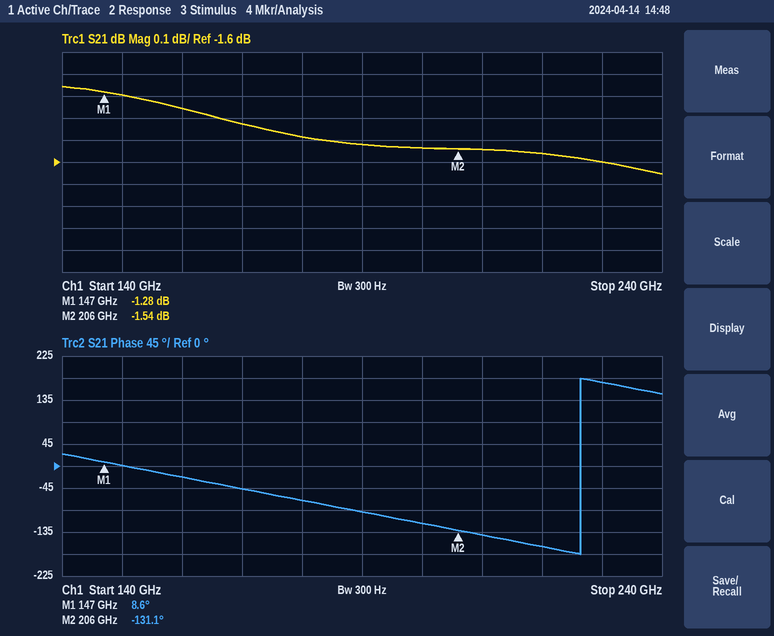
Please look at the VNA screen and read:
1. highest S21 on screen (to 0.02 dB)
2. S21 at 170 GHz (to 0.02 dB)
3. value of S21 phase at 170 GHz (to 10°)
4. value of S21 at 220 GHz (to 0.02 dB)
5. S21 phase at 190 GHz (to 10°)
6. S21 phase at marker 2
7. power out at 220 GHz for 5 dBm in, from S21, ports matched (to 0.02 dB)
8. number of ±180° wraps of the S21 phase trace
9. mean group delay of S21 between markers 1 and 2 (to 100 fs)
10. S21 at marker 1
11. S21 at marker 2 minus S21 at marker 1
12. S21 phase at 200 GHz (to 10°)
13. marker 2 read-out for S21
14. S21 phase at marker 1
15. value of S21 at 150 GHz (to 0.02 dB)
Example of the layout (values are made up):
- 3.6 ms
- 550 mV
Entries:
- -1.26 dB
- -1.42 dB
- -50°
- -1.56 dB
- -90°
- -131.1°
- 3.44 dBm
- 1
- 6.6 ps
- -1.28 dB
- -0.26 dB
- -120°
- -1.54 dB
- 8.6°
- -1.30 dB
